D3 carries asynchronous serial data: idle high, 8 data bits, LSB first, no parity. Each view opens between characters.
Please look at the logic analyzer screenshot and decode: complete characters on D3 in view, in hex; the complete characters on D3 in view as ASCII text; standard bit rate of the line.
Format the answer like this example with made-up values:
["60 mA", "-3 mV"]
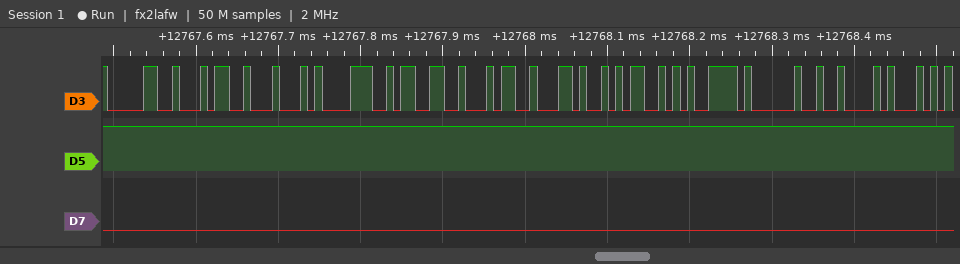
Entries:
["30, 34, 44, 38, 33, 34, 2C, 4D, 79, 20, 42", "\"04D834,My B\"", "115200 baud"]
